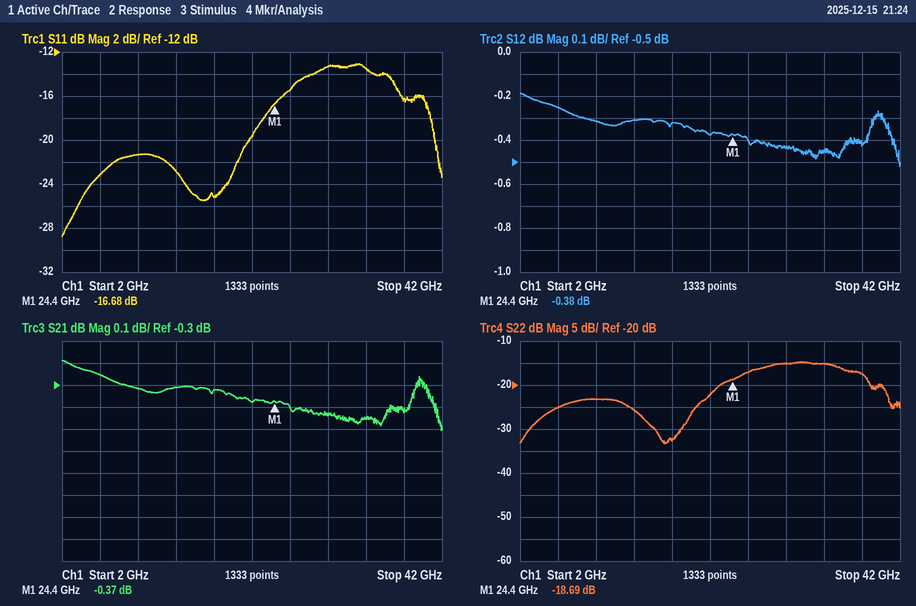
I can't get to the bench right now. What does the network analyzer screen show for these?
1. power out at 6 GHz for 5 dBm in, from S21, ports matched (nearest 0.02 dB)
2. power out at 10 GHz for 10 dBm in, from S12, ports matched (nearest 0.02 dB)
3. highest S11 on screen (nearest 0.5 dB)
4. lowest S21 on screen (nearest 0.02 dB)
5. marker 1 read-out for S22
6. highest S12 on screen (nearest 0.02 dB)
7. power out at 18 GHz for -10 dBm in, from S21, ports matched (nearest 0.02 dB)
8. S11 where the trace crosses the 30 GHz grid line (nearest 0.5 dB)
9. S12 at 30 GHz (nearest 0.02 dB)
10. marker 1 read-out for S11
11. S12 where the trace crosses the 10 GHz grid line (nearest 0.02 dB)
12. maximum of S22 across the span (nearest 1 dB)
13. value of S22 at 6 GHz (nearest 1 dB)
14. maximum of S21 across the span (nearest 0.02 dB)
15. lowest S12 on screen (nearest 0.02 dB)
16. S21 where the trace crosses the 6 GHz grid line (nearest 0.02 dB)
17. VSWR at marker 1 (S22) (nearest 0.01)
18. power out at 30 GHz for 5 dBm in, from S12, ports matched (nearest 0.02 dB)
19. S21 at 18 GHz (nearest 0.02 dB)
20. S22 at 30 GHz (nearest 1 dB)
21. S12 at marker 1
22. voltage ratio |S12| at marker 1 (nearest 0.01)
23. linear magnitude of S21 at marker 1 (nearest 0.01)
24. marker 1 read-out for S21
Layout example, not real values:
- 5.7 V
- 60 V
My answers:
- 4.74 dBm
- 9.68 dBm
- -13.0 dB
- -0.50 dB
- -18.69 dB
- -0.18 dB
- -10.32 dBm
- -13.5 dB
- -0.44 dB
- -16.68 dB
- -0.32 dB
- -15 dB
- -25 dB
- -0.18 dB
- -0.52 dB
- -0.26 dB
- 1.26
- 4.56 dBm
- -0.32 dB
- -15 dB
- -0.38 dB
- 0.96
- 0.96
- -0.37 dB
